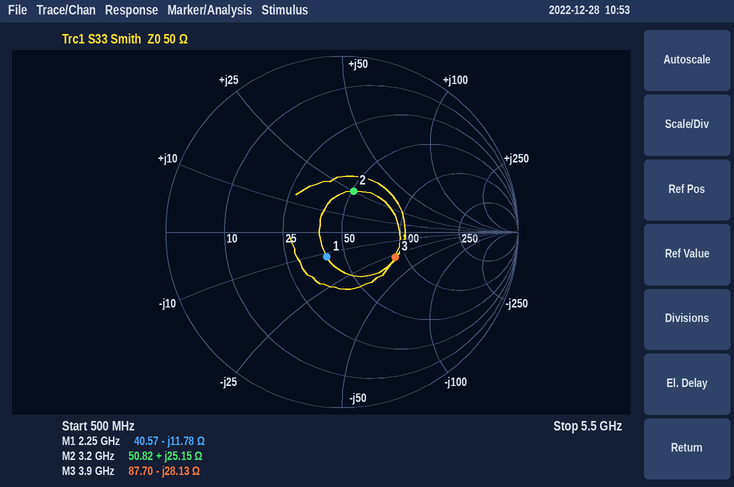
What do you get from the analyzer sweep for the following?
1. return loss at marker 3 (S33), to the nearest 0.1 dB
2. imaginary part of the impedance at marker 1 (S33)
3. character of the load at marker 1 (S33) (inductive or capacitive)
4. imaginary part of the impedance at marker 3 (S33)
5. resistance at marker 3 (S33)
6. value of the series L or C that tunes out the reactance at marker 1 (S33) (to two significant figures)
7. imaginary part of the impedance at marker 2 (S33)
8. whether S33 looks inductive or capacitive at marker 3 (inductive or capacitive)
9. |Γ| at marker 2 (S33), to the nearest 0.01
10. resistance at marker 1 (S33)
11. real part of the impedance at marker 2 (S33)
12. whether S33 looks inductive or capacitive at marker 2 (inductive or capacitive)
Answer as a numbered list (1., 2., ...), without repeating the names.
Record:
1. 9.5 dB
2. -11.78 Ω
3. capacitive
4. -28.13 Ω
5. 87.70 Ω
6. 830 pH
7. +25.15 Ω
8. capacitive
9. 0.24
10. 40.57 Ω
11. 50.82 Ω
12. inductive
